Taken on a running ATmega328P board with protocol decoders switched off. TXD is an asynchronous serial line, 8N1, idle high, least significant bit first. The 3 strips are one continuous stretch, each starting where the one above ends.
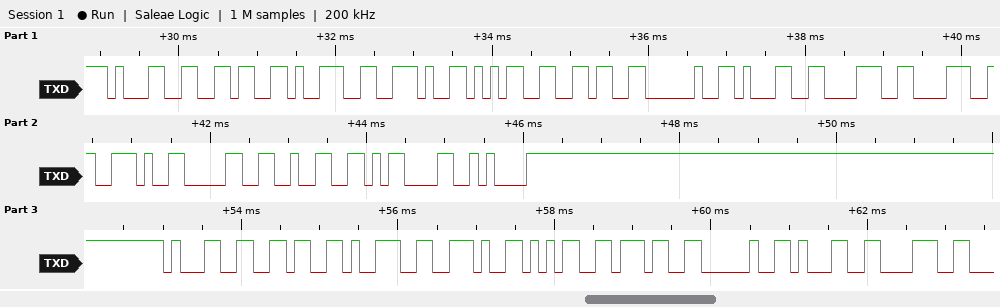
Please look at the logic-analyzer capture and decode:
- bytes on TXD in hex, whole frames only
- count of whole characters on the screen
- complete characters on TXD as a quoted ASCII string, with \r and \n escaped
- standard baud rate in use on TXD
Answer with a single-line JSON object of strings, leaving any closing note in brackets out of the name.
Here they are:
{"bytes on TXD in hex, whole frames only": "0x31 0x36 0x39 0x2E 0x35 0x36 0x20 0x31 0x38 0x38 0x2E 0x30 0x32 0x0D 0x0A 0x31 0x36 0x39 0x2E 0x35 0x37 0x20 0x31 0x38", "count of whole characters on the screen": "24", "complete characters on TXD as a quoted ASCII string, with \\r and \\n escaped": "\"169.56 188.02\\r\\n169.57 18\"", "standard baud rate in use on TXD": "9600 baud"}
